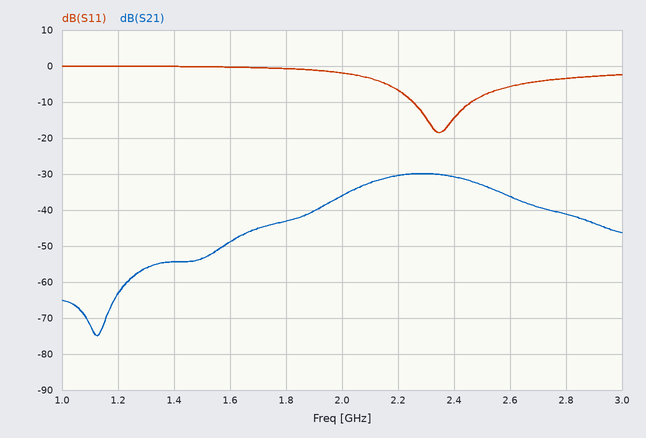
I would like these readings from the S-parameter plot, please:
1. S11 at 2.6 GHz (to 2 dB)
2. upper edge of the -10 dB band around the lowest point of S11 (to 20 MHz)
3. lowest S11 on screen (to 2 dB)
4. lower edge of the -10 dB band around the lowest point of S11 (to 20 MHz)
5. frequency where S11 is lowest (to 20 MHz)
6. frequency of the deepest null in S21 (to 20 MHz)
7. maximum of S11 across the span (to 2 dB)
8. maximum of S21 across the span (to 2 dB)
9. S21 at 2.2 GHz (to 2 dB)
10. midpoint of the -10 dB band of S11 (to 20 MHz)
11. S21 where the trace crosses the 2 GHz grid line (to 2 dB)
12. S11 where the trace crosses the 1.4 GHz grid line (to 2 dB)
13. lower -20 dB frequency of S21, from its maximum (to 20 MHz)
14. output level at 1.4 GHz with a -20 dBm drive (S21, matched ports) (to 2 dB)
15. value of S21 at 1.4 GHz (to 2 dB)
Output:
-6 dB
2.46 GHz
-18 dB
2.26 GHz
2.34 GHz
1.12 GHz
0 dB
-30 dB
-30 dB
2.36 GHz
-36 dB
0 dB
1.58 GHz
-74 dBm
-54 dB
